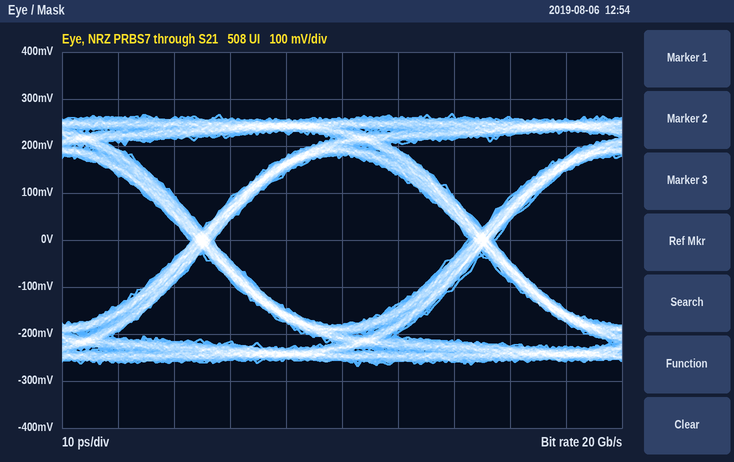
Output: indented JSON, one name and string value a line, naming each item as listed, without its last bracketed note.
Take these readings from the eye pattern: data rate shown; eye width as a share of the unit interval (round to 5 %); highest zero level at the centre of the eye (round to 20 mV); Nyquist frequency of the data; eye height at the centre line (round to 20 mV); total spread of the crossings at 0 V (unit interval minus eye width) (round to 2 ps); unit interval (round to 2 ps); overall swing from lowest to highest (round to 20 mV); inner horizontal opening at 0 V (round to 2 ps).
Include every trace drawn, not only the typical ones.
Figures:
{
  "data rate shown": "20 Gb/s",
  "eye width as a share of the unit interval": "90 %",
  "highest zero level at the centre of the eye": "-180 mV",
  "Nyquist frequency of the data": "10 GHz",
  "eye height at the centre line": "360 mV",
  "total spread of the crossings at 0 V (unit interval minus eye width)": "4 ps",
  "unit interval": "50 ps",
  "overall swing from lowest to highest": "540 mV",
  "inner horizontal opening at 0 V": "46 ps"
}
